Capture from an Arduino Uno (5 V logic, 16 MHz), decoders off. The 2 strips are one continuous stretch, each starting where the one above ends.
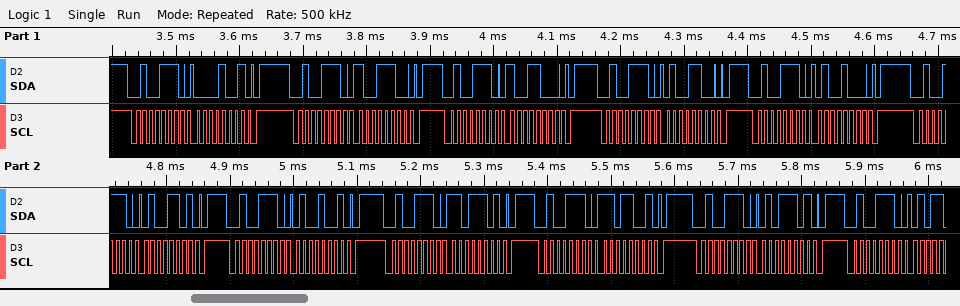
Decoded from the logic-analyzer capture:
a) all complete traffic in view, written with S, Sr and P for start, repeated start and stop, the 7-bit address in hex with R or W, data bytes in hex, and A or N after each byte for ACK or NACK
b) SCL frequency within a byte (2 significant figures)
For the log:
S 27W A 09 A P S 27W A 9C A P S 27W A 98 A P S 27W A 4C A P S 27W A 48 A P S 27W A 4D A P S 27W A 49 A P S 27W A DD A P S 27W A D9 A P S 27W A 5D A P S 27W A
100 kHz
